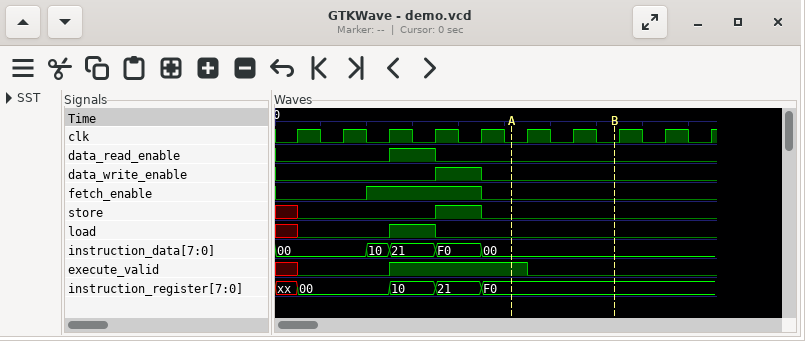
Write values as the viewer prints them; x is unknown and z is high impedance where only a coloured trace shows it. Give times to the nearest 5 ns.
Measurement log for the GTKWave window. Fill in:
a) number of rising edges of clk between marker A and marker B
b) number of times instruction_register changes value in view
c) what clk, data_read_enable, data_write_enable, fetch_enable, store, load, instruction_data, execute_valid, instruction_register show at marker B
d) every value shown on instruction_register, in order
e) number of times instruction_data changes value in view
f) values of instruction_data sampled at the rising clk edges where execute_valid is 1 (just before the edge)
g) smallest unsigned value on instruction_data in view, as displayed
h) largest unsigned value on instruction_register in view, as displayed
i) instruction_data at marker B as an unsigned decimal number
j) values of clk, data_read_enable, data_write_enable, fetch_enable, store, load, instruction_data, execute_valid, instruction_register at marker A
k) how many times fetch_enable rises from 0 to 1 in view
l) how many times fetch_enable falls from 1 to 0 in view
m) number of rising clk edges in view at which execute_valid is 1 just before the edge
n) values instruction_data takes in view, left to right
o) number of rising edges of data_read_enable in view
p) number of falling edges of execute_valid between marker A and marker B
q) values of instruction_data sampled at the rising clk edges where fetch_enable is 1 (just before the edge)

2
4
clk=0, data_read_enable=0, data_write_enable=0, fetch_enable=0, store=0, load=0, instruction_data=00, execute_valid=0, instruction_register=F0
xx, 00, 10, 21, F0
4
21, F0, 00
00
F0
0
clk=0, data_read_enable=0, data_write_enable=0, fetch_enable=0, store=0, load=0, instruction_data=00, execute_valid=1, instruction_register=F0
1
1
3
00, 10, 21, F0, 00
1
1
10, 21, F0
